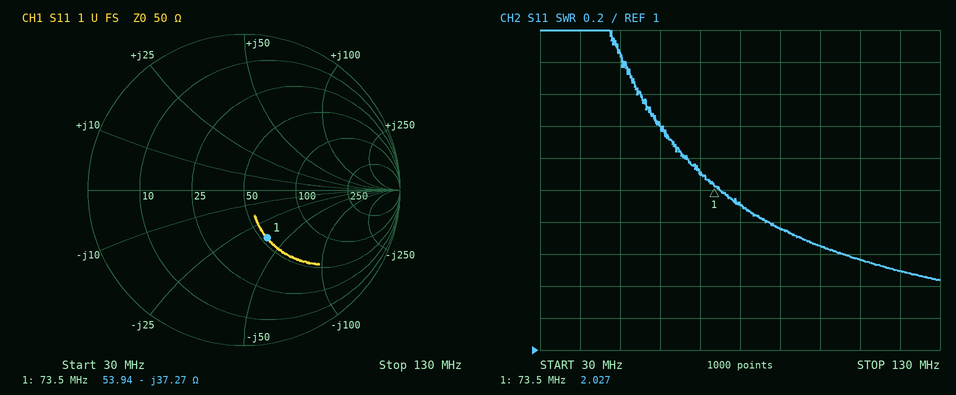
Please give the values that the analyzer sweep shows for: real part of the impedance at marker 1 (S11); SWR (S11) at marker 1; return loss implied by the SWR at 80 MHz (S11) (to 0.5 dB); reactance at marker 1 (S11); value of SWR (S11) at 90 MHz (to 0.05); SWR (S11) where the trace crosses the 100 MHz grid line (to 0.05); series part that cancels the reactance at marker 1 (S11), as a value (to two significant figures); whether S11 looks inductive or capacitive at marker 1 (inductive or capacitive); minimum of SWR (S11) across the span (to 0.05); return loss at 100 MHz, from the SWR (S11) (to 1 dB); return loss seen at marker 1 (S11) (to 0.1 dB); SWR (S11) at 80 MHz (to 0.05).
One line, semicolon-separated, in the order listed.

53.94 Ω; 2.027; 10.0 dB; -37.27 Ω; 1.75; 1.65; 81 nH; capacitive; 1.45; 12 dB; 9.4 dB; 1.90
